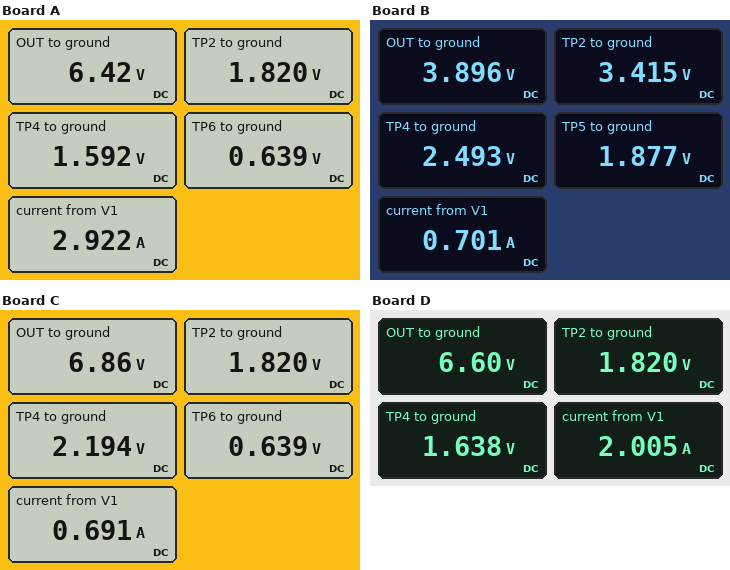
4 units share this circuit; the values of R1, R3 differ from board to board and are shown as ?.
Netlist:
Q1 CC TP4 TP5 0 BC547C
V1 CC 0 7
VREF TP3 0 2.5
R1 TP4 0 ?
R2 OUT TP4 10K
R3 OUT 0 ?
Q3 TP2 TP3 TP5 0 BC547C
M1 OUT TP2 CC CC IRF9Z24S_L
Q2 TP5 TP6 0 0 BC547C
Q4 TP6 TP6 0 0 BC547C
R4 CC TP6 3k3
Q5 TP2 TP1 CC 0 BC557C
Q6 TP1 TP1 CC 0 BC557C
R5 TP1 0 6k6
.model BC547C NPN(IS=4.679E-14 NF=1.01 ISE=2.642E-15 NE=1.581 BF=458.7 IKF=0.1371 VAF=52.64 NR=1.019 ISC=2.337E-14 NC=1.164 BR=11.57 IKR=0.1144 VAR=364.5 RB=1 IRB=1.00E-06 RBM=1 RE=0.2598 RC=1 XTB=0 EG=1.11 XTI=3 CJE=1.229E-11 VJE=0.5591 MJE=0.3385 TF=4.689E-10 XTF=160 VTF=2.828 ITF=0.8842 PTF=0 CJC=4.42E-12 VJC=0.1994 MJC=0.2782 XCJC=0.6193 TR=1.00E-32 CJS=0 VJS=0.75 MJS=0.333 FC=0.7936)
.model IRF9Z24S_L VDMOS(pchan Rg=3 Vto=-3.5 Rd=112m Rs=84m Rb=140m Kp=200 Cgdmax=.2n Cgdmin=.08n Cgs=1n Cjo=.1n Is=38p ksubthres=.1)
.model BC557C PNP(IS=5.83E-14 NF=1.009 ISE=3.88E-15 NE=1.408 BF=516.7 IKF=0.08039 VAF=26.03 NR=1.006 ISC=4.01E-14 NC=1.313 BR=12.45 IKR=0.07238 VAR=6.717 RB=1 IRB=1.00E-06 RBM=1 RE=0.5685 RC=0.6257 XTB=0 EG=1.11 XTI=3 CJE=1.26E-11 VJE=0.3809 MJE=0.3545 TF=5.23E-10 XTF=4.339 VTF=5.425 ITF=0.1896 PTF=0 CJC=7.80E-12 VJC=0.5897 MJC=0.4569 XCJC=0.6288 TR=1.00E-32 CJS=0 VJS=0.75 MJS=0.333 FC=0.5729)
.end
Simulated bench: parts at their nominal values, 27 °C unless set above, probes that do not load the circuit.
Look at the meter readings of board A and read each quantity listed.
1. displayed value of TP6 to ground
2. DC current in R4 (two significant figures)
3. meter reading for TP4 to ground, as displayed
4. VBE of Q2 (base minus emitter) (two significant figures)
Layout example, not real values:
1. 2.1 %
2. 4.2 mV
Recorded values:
1. 0.639 V
2. 1.9 mA
3. 1.592 V
4. 640 mV
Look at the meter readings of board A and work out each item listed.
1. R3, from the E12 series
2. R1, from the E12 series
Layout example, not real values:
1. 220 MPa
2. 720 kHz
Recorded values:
1. 2.2 Ω
2. 3.3 kΩ
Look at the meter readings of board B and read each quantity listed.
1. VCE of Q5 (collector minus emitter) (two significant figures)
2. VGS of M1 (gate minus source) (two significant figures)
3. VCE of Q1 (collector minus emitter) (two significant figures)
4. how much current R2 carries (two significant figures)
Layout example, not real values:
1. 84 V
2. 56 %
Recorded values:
1. -3.6 V
2. -3.6 V
3. 5.1 V
4. 140 µA
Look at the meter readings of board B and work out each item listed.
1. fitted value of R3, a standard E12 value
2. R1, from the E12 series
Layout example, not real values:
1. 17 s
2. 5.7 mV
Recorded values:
1. 5.6 Ω
2. 18 kΩ
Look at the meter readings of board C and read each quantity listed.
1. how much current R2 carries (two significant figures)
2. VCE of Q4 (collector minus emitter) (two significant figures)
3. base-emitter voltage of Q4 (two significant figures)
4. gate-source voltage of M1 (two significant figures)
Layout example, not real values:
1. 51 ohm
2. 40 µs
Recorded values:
1. 470 µA
2. 640 mV
3. 640 mV
4. -5.2 V
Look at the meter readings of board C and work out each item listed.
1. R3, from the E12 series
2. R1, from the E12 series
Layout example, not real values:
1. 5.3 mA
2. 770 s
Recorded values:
1. 10 Ω
2. 4.7 kΩ
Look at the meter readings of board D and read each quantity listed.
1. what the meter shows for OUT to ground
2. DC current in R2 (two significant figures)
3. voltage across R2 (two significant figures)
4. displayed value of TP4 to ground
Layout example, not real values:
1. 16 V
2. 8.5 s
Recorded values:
1. 6.60 V
2. 500 µA
3. 5.0 V
4. 1.638 V
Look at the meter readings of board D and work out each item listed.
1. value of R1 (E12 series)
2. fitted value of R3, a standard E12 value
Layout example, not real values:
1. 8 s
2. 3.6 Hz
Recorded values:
1. 3.3 kΩ
2. 3.3 Ω
